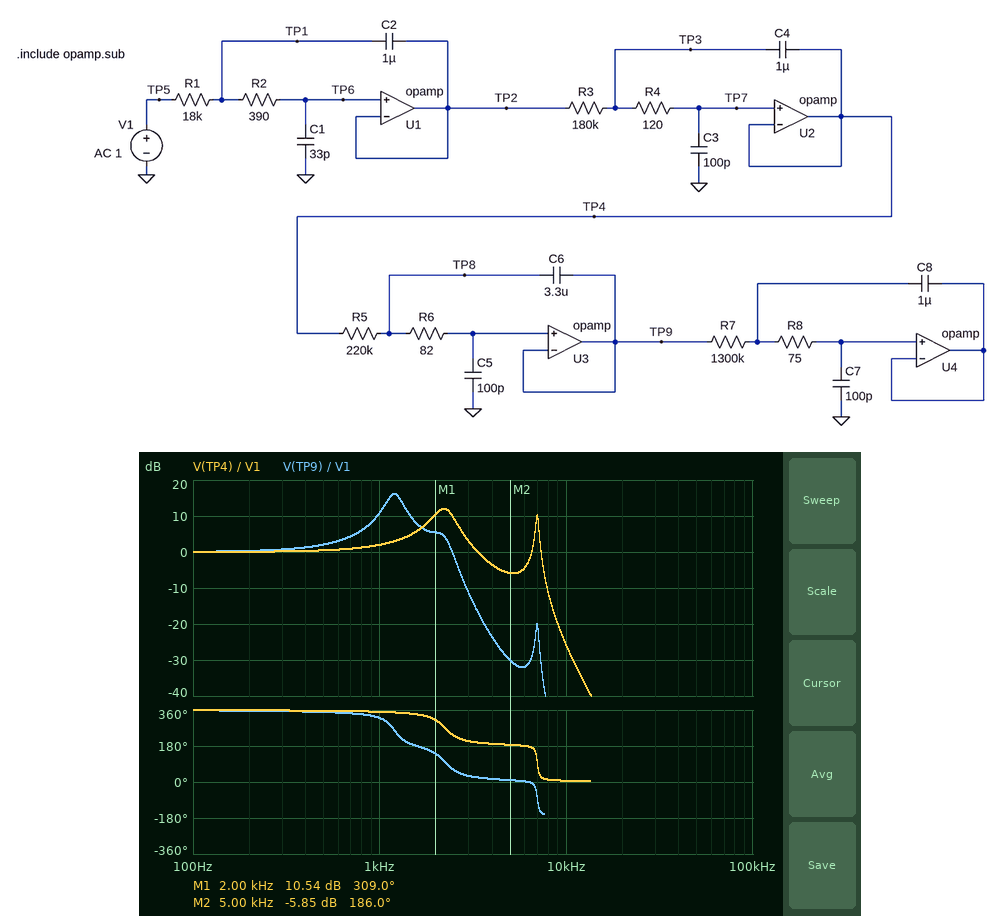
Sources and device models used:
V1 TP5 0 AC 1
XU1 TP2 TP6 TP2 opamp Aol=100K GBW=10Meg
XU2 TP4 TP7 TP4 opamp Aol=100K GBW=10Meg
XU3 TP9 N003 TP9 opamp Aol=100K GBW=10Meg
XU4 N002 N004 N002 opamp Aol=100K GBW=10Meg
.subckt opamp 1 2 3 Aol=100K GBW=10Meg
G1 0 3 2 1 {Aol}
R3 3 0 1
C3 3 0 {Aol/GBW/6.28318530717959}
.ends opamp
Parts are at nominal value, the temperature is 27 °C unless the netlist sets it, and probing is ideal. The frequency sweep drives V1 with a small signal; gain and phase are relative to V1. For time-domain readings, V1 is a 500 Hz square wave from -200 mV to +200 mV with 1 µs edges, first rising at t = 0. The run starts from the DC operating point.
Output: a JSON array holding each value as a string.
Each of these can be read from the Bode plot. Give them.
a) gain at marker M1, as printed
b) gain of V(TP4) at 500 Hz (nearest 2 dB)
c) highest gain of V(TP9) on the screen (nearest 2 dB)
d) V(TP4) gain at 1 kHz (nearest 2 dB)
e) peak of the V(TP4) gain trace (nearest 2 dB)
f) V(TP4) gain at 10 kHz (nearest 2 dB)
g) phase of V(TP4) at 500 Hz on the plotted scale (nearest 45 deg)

["10.54 dB", "0 dB", "16 dB", "2 dB", "12 dB", "-26 dB", "360 deg"]
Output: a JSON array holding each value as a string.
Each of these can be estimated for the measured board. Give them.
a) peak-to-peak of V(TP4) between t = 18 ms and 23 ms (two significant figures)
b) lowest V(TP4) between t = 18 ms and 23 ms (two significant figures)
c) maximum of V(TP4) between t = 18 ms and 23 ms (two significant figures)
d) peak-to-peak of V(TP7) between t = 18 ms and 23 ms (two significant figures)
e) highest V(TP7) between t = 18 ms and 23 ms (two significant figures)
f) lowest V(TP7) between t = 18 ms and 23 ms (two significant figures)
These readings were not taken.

["930 mV", "-470 mV", "470 mV", "930 mV", "470 mV", "-470 mV"]
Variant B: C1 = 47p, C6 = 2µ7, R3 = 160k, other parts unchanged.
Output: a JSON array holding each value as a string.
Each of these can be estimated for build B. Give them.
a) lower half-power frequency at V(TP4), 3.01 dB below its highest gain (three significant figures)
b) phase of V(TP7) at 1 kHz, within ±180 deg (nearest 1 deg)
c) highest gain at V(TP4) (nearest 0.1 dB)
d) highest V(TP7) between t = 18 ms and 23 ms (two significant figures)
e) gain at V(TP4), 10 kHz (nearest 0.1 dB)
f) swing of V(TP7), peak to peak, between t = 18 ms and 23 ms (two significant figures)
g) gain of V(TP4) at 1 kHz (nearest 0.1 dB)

["2.03 kHz", "-8 deg", "12.9 dB", "540 mV", "-27.6 dB", "1.1 V", "1.8 dB"]
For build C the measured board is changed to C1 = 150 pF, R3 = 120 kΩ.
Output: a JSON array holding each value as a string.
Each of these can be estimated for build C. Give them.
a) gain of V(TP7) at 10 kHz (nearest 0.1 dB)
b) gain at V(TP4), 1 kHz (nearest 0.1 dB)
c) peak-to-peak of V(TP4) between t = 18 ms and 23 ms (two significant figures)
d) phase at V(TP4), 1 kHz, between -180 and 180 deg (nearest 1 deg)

["-34.4 dB", "1.7 dB", "1.5 V", "-7 deg"]
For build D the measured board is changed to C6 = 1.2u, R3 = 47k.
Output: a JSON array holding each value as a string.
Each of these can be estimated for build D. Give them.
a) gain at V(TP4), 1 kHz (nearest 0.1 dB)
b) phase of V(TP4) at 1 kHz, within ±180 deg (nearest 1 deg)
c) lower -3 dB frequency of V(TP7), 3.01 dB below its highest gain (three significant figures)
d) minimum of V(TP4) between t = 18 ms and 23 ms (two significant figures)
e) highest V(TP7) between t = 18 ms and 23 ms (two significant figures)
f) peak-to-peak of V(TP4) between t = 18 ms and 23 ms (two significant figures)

["0.6 dB", "-2 deg", "6.85 kHz", "-890 mV", "890 mV", "1.8 V"]
